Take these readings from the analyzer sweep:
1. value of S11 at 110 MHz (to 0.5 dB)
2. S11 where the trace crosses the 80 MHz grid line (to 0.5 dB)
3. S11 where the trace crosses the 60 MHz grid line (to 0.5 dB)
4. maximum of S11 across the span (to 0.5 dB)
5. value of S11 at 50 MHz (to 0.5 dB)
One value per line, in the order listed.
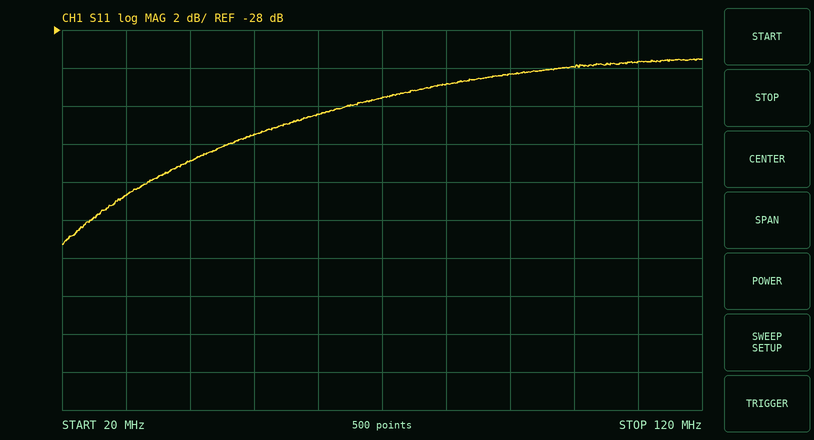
-29.5 dB
-31.0 dB
-32.5 dB
-29.5 dB
-33.5 dB
